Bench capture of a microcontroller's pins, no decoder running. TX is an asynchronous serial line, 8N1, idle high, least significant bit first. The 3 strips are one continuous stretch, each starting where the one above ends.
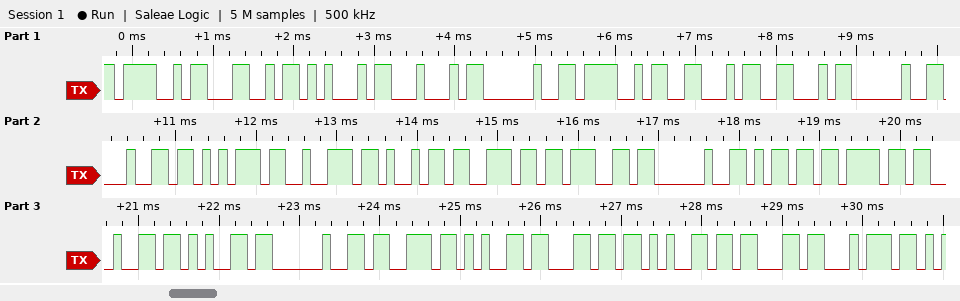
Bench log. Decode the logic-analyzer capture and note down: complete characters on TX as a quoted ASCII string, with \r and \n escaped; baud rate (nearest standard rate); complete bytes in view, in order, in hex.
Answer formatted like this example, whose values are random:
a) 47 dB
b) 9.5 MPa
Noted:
a) "OLED OFF during mode select"
b) 9600 baud
c) 4F 4C 45 44 20 4F 46 46 20 64 75 72 69 6E 67 20 6D 6F 64 65 20 73 65 6C 65 63 74
